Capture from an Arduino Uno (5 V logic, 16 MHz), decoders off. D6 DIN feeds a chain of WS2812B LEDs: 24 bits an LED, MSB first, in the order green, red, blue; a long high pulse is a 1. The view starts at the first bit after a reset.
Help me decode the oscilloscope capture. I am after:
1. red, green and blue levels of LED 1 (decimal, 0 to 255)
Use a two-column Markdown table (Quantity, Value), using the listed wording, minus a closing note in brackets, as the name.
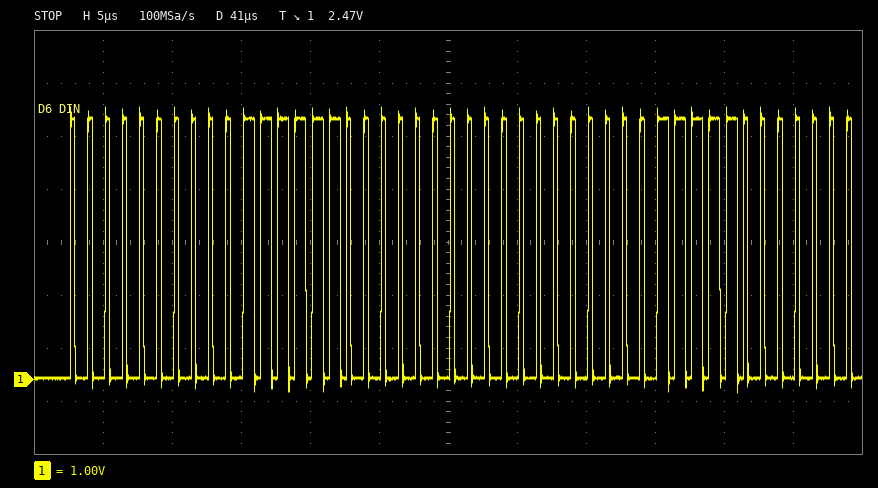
| Quantity | Value |
|---|---|
| red, green and blue levels of LED 1 | 63, 0, 0 |
